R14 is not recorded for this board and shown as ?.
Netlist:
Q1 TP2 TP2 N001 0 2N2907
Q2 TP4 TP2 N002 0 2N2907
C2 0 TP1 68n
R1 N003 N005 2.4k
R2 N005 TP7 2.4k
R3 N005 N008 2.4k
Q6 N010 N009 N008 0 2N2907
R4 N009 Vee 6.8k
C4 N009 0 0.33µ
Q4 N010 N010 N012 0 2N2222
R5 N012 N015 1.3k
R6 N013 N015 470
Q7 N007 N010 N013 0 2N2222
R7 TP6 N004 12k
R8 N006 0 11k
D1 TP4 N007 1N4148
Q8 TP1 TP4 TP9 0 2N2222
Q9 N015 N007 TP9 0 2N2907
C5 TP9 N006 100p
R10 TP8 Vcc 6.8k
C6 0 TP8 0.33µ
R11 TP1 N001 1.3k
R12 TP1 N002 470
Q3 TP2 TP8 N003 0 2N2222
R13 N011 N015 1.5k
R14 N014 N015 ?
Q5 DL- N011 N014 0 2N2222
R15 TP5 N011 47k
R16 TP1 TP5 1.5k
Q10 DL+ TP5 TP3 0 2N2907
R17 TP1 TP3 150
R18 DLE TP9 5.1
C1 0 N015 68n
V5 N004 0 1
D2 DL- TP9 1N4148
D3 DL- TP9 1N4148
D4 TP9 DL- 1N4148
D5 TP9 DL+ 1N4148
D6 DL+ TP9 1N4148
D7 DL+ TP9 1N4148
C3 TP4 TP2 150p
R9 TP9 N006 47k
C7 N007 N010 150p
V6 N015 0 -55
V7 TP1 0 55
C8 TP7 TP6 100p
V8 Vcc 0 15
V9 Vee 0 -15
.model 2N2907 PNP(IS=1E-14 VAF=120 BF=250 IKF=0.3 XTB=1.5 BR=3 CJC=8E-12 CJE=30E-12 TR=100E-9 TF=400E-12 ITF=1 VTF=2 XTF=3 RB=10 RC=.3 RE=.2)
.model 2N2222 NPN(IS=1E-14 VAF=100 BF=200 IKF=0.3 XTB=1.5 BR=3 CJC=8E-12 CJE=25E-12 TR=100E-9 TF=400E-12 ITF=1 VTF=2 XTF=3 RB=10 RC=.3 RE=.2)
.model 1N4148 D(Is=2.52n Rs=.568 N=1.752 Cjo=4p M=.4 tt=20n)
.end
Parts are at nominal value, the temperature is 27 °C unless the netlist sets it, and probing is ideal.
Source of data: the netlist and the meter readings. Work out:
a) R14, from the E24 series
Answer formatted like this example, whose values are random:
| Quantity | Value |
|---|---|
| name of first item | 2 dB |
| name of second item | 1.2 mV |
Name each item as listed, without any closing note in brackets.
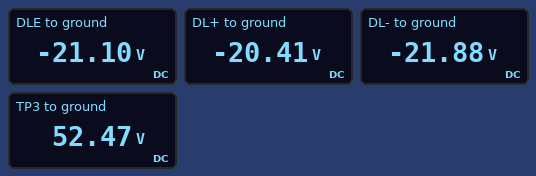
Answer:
| Quantity | Value |
|---|---|
| R14, from the E24 series | 47 Ω |
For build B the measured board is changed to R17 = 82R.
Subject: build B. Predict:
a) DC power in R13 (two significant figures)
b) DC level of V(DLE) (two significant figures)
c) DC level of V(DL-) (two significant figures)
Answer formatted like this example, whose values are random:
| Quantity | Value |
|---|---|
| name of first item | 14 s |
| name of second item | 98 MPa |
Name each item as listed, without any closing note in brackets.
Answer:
| Quantity | Value |
|---|---|
| DC power in R13 | 6.1 mW |
| DC level of V(DLE) | -11 V |
| DC level of V(DL-) | -12 V |
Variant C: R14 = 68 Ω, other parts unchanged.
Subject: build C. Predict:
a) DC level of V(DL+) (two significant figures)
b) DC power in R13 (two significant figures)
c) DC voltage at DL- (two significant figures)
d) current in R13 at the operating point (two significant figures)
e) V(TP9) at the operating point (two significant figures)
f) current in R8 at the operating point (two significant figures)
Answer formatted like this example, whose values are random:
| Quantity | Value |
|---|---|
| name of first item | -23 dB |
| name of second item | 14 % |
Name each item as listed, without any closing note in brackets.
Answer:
| Quantity | Value |
|---|---|
| DC level of V(DL+) | -10 V |
| DC power in R13 | 6.4 mW |
| DC voltage at DL- | -12 V |
| current in R13 at the operating point | 2.1 mA |
| V(TP9) at the operating point | -11 V |
| current in R8 at the operating point | 190 µA |
